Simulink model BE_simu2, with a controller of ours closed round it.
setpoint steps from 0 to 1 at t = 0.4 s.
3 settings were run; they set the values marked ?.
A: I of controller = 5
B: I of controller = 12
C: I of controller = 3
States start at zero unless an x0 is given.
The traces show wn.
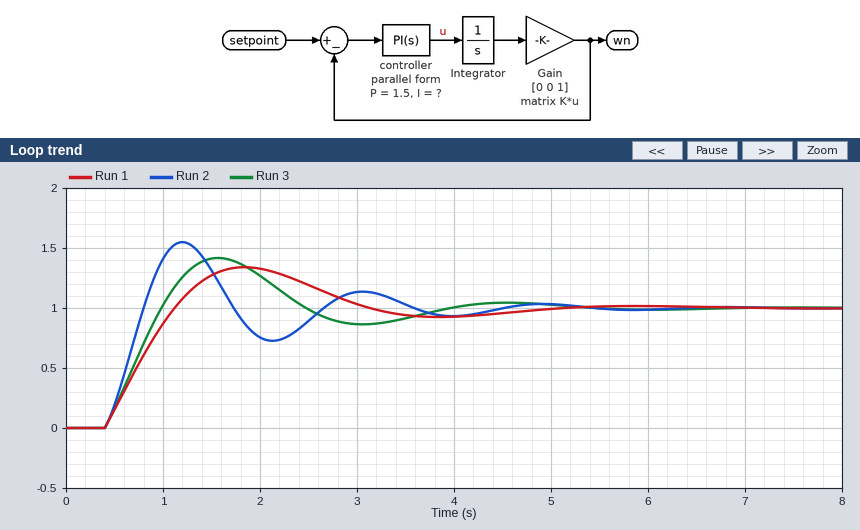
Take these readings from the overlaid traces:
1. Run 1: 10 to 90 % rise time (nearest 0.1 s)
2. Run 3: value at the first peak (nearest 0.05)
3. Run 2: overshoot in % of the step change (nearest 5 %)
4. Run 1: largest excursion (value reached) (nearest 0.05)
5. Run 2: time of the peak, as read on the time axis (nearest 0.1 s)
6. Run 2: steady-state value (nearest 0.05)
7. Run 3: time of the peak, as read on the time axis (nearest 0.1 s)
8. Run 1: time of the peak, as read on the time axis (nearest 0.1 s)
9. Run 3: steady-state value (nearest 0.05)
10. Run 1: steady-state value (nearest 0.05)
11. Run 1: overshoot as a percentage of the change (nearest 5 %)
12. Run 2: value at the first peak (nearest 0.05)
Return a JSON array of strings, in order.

["0.6 s", "1.40", "55 %", "1.35", "1.2 s", "1.00", "1.6 s", "1.8 s", "1.00", "1.00", "35 %", "1.55"]
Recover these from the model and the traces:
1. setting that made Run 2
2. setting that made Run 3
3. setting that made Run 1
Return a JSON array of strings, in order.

["B", "A", "C"]
